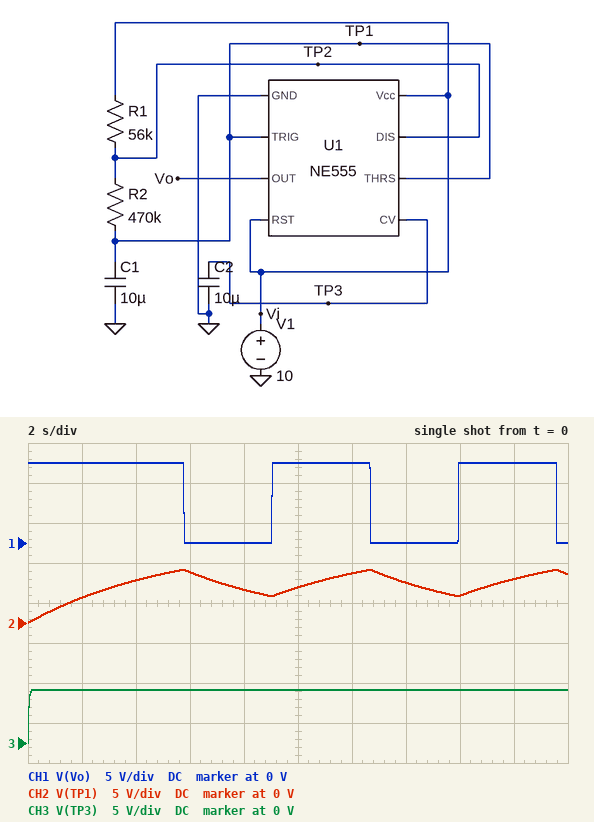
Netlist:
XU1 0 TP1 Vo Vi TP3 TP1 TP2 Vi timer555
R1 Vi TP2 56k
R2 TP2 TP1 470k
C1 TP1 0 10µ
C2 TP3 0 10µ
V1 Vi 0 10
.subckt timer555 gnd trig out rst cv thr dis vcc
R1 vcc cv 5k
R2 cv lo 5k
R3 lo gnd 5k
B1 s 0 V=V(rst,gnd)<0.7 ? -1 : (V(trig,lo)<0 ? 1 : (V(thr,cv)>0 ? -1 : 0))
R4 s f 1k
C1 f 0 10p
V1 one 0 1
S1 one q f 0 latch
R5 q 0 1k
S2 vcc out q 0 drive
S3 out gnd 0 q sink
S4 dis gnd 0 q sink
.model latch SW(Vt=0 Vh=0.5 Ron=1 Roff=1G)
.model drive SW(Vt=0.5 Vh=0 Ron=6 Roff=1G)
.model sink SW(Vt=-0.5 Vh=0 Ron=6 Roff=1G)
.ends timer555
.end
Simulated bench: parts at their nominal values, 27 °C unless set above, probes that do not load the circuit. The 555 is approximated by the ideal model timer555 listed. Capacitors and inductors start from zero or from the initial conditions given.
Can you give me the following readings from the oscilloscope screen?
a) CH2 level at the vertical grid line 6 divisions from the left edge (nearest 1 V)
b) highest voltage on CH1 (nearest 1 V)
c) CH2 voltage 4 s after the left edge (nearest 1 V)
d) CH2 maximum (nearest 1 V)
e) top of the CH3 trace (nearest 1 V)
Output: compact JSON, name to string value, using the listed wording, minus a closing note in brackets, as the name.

{"CH2 level at the vertical grid line 6 divisions from the left edge": "6 V", "highest voltage on CH1": "10 V", "CH2 voltage 4 s after the left edge": "5 V", "CH2 maximum": "7 V", "top of the CH3 trace": "7 V"}
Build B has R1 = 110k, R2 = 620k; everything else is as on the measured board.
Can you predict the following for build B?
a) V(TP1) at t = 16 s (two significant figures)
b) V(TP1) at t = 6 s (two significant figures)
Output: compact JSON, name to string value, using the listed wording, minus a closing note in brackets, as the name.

{"V(TP1) at t = 16 s": "6.0 V", "V(TP1) at t = 6 s": "5.6 V"}
